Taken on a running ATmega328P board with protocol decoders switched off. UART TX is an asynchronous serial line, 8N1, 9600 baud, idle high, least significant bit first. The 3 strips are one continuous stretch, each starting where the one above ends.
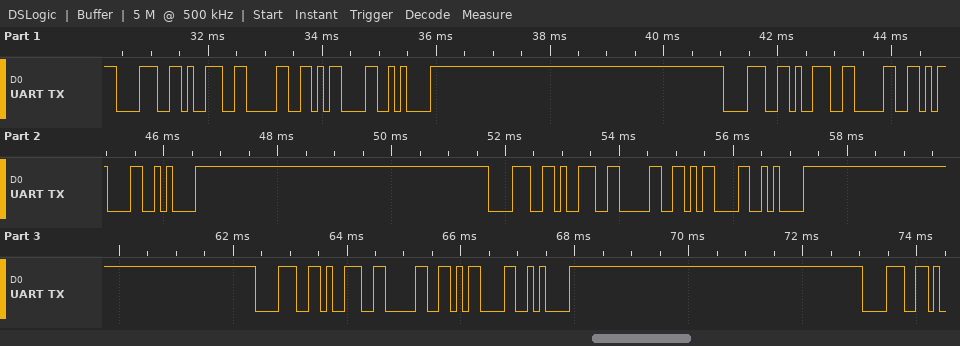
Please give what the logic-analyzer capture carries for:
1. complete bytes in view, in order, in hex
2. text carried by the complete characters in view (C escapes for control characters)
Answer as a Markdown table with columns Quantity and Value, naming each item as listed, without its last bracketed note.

| Quantity | Value |
|---|---|
| complete bytes in view, in order, in hex | 38 39 30 0D 0A 38 39 30 0D 0A 38 39 30 0D 0A 38 39 30 0D 0A 38 |
| text carried by the complete characters in view | "890\r\n890\r\n890\r\n890\r\n8" |
